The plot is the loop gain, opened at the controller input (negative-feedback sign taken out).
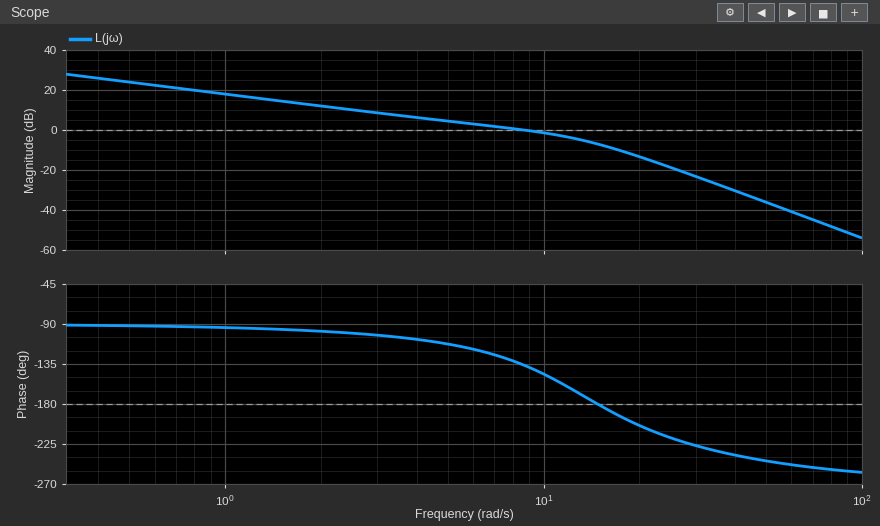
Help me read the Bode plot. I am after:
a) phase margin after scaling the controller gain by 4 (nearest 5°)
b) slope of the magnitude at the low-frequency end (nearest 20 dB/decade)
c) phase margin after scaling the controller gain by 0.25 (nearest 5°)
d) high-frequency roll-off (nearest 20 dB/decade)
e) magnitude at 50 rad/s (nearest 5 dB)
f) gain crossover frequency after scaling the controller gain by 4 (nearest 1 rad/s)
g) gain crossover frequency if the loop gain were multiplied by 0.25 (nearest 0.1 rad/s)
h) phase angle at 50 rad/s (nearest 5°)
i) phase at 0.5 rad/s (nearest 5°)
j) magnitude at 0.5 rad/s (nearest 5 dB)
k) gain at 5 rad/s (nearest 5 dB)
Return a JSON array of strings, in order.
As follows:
["-20°", "-20 dB/decade", "80°", "-60 dB/decade", "-35 dB", "19 rad/s", "2.0 rad/s", "-245°", "-90°", "25 dB", "5 dB"]
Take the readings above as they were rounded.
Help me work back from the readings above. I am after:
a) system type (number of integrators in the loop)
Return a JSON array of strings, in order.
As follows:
["1"]
